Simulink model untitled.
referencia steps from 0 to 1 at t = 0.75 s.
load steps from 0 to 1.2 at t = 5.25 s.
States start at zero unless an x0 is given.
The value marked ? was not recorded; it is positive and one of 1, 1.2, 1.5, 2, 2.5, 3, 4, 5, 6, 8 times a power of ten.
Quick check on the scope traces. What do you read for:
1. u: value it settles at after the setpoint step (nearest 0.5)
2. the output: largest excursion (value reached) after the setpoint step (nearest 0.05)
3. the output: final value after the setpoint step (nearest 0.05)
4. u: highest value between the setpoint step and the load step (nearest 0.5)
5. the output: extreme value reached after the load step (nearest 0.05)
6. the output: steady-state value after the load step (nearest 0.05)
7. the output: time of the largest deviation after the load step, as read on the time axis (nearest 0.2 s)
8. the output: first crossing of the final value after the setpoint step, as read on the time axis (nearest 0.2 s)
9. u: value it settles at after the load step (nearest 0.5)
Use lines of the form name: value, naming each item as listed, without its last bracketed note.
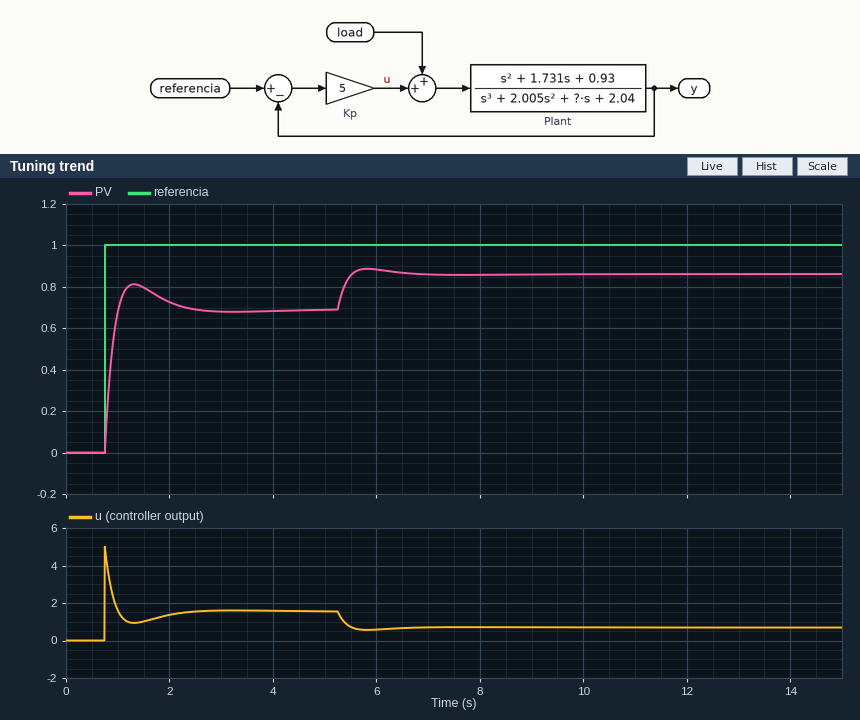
u: value it settles at after the setpoint step: 1.5
the output: largest excursion (value reached) after the setpoint step: 0.80
the output: final value after the setpoint step: 0.70
u: highest value between the setpoint step and the load step: 5.0
the output: extreme value reached after the load step: 0.90
the output: steady-state value after the load step: 0.85
the output: time of the largest deviation after the load step, as read on the time axis: 5.8 s
the output: first crossing of the final value after the setpoint step, as read on the time axis: 1.0 s
u: value it settles at after the load step: 0.5
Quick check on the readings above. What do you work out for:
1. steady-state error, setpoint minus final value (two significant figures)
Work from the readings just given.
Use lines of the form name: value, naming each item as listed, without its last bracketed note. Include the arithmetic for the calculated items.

steady-state error, setpoint minus final value: 1 - 0.7 = 0.30
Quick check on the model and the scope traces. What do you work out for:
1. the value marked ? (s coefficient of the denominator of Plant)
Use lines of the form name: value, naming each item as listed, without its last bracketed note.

the value marked ?: 4
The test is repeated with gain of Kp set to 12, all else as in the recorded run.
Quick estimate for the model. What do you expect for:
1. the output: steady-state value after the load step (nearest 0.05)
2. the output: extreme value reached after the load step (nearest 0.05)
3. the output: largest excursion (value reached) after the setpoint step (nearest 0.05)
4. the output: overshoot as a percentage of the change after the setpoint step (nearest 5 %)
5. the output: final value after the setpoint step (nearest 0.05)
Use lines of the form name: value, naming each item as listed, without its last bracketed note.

the output: steady-state value after the load step: 0.95
the output: extreme value reached after the load step: 0.95
the output: largest excursion (value reached) after the setpoint step: 0.95
the output: overshoot as a percentage of the change after the setpoint step: 10 %
the output: final value after the setpoint step: 0.85
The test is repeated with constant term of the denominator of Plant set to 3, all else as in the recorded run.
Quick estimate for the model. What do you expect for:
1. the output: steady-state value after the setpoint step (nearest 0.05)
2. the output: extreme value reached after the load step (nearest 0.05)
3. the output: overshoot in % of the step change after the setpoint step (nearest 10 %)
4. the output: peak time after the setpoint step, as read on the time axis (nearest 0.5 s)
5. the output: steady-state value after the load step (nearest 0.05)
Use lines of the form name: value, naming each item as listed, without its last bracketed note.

the output: steady-state value after the setpoint step: 0.60
the output: extreme value reached after the load step: 0.80
the output: overshoot in % of the step change after the setpoint step: 30 %
the output: peak time after the setpoint step, as read on the time axis: 1.5 s
the output: steady-state value after the load step: 0.75
